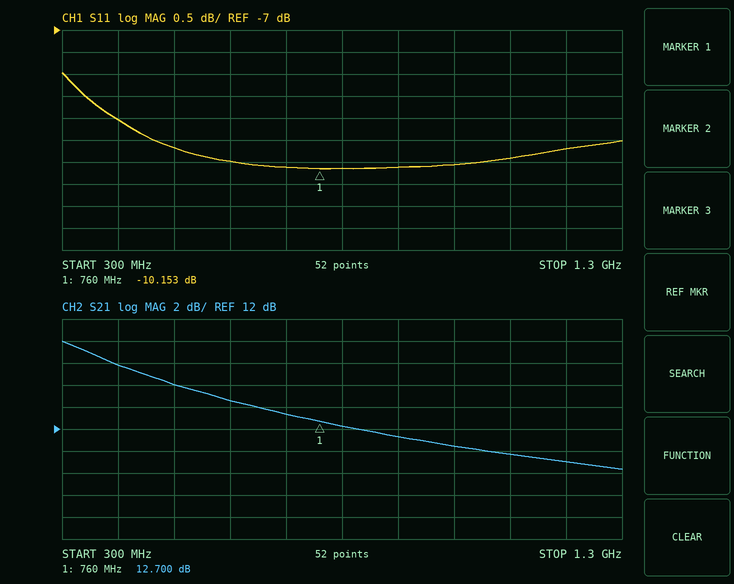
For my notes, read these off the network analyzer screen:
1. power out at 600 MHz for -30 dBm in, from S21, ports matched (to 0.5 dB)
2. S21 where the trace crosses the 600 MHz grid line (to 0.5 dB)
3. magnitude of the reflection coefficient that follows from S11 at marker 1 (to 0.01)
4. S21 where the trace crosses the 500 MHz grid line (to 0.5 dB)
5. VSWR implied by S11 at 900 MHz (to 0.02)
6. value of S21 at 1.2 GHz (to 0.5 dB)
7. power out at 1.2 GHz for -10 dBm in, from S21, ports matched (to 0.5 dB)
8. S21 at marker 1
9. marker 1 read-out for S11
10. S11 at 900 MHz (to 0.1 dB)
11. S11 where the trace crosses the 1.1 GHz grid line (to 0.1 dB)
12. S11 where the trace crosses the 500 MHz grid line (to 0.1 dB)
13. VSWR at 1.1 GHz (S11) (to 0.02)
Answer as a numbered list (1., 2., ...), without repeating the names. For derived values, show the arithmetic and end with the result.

1. -30 dBm + (14.5 dB) = -15.5 dBm
2. 14.5 dB
3. 10^(-10.153/20) ≈ 0.31
4. 16.0 dB
5. |Γ| = 10^(-10.1/20) = 0.3126; VSWR = (1 + 0.3126)/(1 − 0.3126) ≈ 1.91, so 1.90 to the nearest 0.02
6. 9.0 dB
7. -10 dBm + (9.0 dB) = -1.0 dBm
8. 12.700 dB
9. -10.153 dB
10. -10.1 dB
11. -9.9 dB
12. -9.7 dB
13. |Γ| = 10^(-9.9/20) = 0.3199; VSWR = (1 + 0.3199)/(1 − 0.3199) ≈ 1.94
